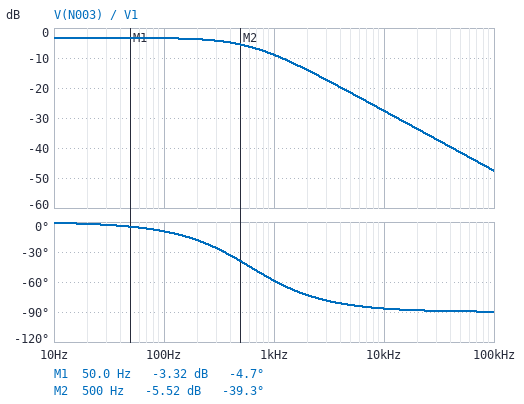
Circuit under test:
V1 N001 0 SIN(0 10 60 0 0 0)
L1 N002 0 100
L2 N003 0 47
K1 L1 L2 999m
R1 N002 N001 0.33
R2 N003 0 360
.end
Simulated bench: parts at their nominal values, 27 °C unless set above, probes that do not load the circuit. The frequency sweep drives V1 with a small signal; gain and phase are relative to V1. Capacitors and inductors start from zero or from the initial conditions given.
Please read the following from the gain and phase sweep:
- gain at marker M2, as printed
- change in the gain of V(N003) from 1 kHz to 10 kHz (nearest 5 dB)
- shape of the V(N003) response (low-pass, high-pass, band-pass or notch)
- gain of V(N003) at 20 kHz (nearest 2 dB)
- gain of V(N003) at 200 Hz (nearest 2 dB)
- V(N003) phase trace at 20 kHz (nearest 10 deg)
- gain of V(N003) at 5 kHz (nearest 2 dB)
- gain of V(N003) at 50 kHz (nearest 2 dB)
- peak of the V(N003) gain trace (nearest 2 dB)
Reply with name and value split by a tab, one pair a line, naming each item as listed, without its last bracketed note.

gain at marker M2, as printed	-5.52 dB
change in the gain of V(N003) from 1 kHz to 10 kHz	-20 dB
shape of the V(N003) response	low-pass
gain of V(N003) at 20 kHz	-34 dB
gain of V(N003) at 200 Hz	-4 dB
V(N003) phase trace at 20 kHz	-90 deg
gain of V(N003) at 5 kHz	-22 dB
gain of V(N003) at 50 kHz	-42 dB
peak of the V(N003) gain trace	-4 dB
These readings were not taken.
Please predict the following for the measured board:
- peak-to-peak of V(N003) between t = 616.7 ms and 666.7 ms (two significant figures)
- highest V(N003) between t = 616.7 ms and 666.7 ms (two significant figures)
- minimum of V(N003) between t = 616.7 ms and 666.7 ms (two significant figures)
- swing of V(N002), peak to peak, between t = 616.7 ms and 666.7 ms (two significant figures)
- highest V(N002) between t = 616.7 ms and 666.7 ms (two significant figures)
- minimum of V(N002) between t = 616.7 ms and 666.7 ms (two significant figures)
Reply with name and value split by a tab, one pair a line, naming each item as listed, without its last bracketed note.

peak-to-peak of V(N003) between t = 616.7 ms and 666.7 ms	14 V
highest V(N003) between t = 616.7 ms and 666.7 ms	6.8 V
minimum of V(N003) between t = 616.7 ms and 666.7 ms	-6.8 V
swing of V(N002), peak to peak, between t = 616.7 ms and 666.7 ms	20 V
highest V(N002) between t = 616.7 ms and 666.7 ms	10 V
minimum of V(N002) between t = 616.7 ms and 666.7 ms	-10 V
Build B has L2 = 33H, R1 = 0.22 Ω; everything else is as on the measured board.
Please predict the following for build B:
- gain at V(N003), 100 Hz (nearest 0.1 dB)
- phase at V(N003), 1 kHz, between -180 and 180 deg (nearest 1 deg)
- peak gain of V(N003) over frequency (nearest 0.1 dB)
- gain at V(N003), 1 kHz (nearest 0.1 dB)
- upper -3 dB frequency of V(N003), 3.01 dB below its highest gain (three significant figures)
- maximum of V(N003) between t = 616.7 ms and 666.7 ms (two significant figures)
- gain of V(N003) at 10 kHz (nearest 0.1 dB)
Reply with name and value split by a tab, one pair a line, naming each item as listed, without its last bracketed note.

gain at V(N003), 100 Hz	-4.9 dB
phase at V(N003), 1 kHz, between -180 and 180 deg	-49 deg
peak gain of V(N003) over frequency	-4.8 dB
gain at V(N003), 1 kHz	-8.5 dB
upper -3 dB frequency of V(N003), 3.01 dB below its highest gain	869 Hz
maximum of V(N003) between t = 616.7 ms and 666.7 ms	5.7 V
gain of V(N003) at 10 kHz	-26.1 dB
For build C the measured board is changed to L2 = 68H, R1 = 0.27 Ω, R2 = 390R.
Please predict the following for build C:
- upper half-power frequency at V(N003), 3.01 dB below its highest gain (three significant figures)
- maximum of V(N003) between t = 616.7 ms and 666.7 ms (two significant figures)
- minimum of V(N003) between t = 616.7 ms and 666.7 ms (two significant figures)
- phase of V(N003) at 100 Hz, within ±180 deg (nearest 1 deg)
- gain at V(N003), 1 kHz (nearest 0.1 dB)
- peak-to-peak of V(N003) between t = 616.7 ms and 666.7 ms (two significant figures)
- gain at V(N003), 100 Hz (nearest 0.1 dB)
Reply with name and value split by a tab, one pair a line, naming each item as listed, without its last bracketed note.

upper half-power frequency at V(N003), 3.01 dB below its highest gain	457 Hz
maximum of V(N003) between t = 616.7 ms and 666.7 ms	8.2 V
minimum of V(N003) between t = 616.7 ms and 666.7 ms	-8.2 V
phase of V(N003) at 100 Hz, within ±180 deg	-12 deg
gain at V(N003), 1 kHz	-9.3 dB
peak-to-peak of V(N003) between t = 616.7 ms and 666.7 ms	16 V
gain at V(N003), 100 Hz	-1.9 dB
